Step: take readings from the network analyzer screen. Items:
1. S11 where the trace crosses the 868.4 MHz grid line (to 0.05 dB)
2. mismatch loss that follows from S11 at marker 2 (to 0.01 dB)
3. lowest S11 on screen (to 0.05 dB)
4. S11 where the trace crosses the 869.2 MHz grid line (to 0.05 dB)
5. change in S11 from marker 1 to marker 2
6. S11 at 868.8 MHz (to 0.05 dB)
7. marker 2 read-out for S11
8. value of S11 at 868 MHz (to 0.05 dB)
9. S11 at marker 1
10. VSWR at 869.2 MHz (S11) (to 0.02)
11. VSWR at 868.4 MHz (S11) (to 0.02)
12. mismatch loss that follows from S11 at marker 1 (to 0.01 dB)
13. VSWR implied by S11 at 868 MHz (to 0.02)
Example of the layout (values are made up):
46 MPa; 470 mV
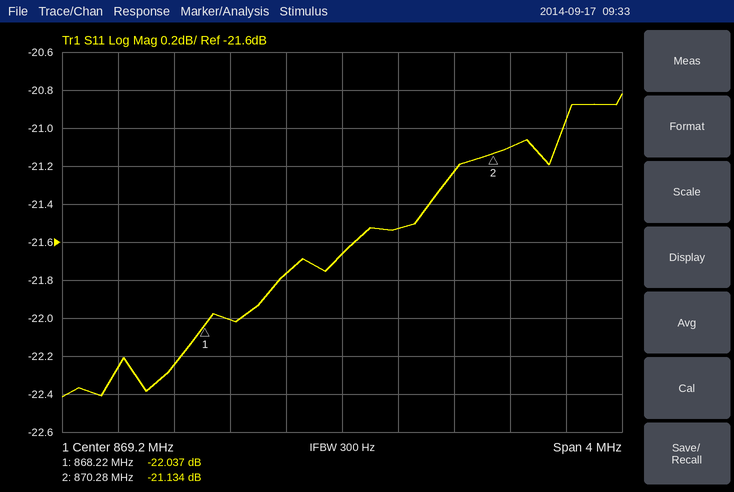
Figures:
-22.00 dB; 0.03 dB; -22.40 dB; -21.65 dB; 0.903 dB; -21.75 dB; -21.134 dB; -22.25 dB; -22.037 dB; 1.18; 1.18; 0.03 dB; 1.16
